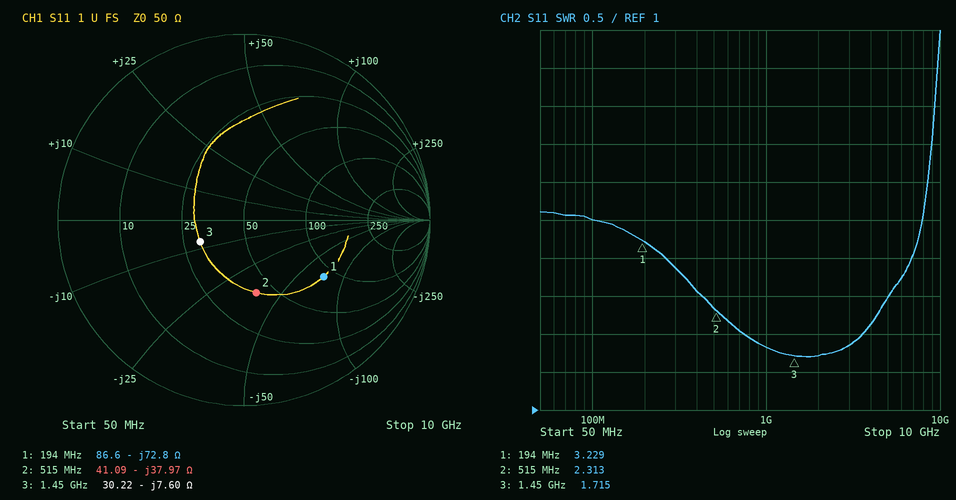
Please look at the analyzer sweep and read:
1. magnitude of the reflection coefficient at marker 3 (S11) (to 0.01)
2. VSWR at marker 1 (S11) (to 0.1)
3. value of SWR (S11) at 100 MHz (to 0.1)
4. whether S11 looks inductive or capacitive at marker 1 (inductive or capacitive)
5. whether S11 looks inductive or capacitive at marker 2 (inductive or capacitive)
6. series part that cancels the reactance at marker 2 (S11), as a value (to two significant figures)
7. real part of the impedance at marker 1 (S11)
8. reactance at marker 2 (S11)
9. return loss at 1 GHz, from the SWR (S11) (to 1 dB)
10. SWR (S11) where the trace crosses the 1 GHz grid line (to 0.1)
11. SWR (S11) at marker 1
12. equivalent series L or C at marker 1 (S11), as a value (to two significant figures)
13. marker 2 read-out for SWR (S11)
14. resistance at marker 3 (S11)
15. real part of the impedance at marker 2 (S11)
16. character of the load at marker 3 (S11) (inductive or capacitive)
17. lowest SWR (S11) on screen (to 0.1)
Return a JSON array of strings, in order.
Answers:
["0.26", "3.2", "3.5", "capacitive", "capacitive", "12 nH", "86.6 Ω", "-37.97 Ω", "11 dB", "1.8", "3.229", "11 pF", "2.313", "30.22 Ω", "41.09 Ω", "capacitive", "1.7"]
